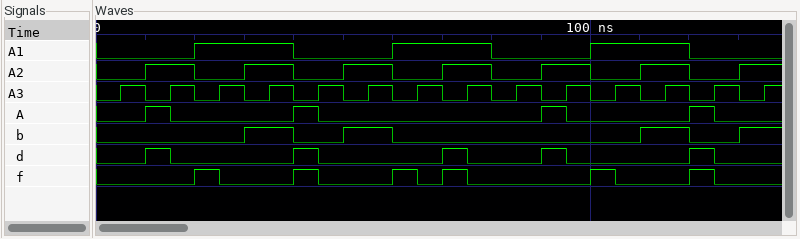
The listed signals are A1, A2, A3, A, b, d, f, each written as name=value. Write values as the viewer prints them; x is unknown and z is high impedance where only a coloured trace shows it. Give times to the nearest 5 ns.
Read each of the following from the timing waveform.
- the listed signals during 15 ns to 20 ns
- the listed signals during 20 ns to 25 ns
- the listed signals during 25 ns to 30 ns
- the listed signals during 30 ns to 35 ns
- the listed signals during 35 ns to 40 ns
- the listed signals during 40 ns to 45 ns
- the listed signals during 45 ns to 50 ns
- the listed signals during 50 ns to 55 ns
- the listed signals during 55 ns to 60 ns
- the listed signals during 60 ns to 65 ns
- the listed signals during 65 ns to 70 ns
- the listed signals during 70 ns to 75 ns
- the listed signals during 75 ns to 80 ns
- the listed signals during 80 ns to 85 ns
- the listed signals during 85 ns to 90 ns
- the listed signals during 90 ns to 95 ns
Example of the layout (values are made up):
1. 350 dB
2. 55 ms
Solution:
1. A1=0, A2=1, A3=1, A=0, b=0, d=0, f=0
2. A1=1, A2=0, A3=0, A=0, b=0, d=0, f=1
3. A1=1, A2=0, A3=1, A=0, b=0, d=0, f=0
4. A1=1, A2=1, A3=0, A=0, b=1, d=0, f=0
5. A1=1, A2=1, A3=1, A=0, b=1, d=0, f=0
6. A1=0, A2=0, A3=0, A=1, b=0, d=1, f=1
7. A1=0, A2=0, A3=1, A=0, b=0, d=0, f=0
8. A1=0, A2=1, A3=0, A=0, b=1, d=0, f=0
9. A1=0, A2=1, A3=1, A=0, b=1, d=0, f=0
10. A1=1, A2=0, A3=0, A=0, b=0, d=0, f=1
11. A1=1, A2=0, A3=1, A=0, b=0, d=0, f=0
12. A1=1, A2=1, A3=0, A=0, b=0, d=1, f=1
13. A1=1, A2=1, A3=1, A=0, b=0, d=0, f=0
14. A1=0, A2=0, A3=0, A=0, b=0, d=0, f=0
15. A1=0, A2=0, A3=1, A=0, b=0, d=0, f=0
16. A1=0, A2=1, A3=0, A=1, b=0, d=1, f=0
